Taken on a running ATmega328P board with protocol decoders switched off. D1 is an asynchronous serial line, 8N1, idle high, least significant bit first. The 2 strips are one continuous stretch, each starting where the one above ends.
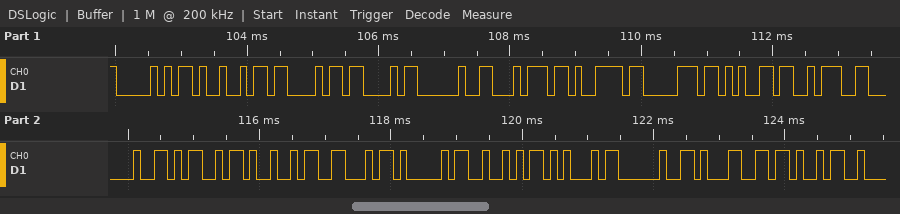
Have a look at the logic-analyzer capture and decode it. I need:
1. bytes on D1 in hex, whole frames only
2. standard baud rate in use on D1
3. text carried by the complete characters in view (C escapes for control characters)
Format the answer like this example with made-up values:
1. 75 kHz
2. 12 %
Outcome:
1. 50 49 43 43 20 74 79 70 65 3A 20 4D 49 46 41 52 45 20 31 4B
2. 9600 baud
3. "PICC type: MIFARE 1K"
